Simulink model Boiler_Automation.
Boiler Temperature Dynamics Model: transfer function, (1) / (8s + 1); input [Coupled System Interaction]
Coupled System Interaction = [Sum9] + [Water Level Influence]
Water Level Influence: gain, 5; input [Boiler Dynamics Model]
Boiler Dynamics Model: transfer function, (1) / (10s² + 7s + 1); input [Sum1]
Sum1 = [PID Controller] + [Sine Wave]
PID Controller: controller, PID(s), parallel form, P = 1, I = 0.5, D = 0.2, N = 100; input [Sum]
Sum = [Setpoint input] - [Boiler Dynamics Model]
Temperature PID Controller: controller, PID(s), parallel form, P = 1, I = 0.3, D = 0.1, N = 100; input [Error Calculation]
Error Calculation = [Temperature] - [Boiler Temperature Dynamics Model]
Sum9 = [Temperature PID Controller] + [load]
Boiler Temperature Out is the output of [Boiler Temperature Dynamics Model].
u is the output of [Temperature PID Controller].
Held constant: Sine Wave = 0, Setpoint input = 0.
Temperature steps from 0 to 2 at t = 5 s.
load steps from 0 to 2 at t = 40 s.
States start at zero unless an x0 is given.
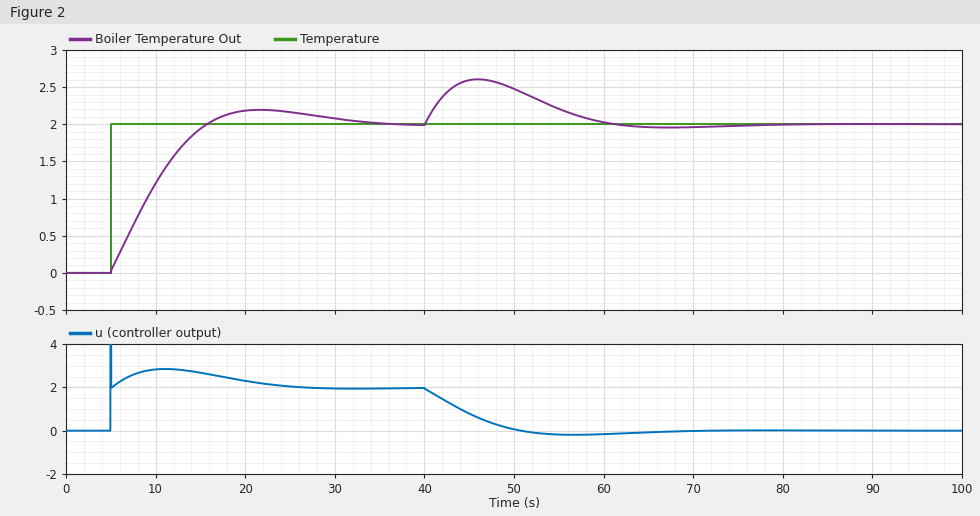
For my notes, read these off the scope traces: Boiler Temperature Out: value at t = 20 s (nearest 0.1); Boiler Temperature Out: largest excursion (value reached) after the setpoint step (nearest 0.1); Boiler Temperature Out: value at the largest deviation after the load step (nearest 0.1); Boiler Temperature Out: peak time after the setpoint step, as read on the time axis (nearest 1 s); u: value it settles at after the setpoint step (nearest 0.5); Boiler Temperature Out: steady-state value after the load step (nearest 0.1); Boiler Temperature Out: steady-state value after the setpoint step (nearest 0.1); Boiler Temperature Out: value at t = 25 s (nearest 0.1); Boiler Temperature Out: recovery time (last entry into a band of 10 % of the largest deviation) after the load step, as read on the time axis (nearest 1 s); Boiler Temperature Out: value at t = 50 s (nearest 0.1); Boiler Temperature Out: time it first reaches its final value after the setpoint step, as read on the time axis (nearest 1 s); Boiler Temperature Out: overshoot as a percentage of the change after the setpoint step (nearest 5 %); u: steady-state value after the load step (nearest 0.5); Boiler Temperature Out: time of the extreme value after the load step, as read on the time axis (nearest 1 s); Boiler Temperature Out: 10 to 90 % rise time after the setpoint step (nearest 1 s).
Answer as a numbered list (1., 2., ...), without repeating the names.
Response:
1. 2.2
2. 2.2
3. 2.6
4. 22 s
5. 2.0
6. 2.0
7. 2.0
8. 2.2
9. 59 s
10. 2.5
11. 16 s
12. 10 %
13. 0.0
14. 46 s
15. 8 s
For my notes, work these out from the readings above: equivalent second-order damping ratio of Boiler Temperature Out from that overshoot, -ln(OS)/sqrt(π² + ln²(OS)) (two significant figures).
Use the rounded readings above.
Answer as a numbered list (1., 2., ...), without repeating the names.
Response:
1. 0.59
